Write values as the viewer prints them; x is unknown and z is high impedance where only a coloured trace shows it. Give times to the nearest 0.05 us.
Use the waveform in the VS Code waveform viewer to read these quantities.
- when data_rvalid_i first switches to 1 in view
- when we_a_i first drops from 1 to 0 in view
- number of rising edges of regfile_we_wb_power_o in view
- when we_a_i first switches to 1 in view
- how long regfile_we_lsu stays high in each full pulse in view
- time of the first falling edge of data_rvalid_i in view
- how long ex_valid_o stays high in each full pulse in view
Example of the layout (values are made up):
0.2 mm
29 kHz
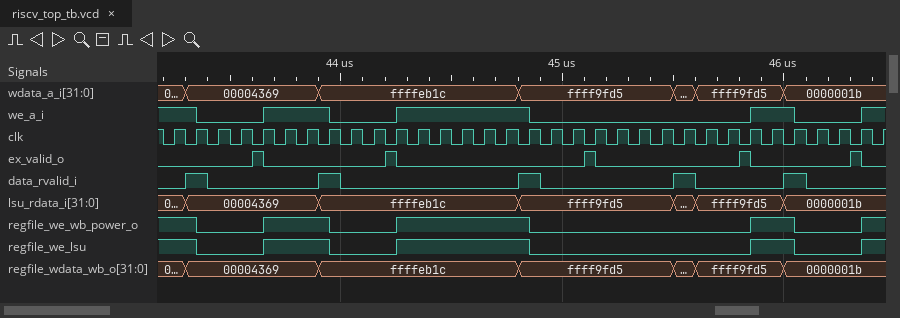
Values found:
43.3 us
43.35 us
4
43.65 us
0.3 us, 0.6 us, 0.2 us
43.4 us
0.05 us, 0.05 us, 0.05 us, 0.05 us, 0.05 us
